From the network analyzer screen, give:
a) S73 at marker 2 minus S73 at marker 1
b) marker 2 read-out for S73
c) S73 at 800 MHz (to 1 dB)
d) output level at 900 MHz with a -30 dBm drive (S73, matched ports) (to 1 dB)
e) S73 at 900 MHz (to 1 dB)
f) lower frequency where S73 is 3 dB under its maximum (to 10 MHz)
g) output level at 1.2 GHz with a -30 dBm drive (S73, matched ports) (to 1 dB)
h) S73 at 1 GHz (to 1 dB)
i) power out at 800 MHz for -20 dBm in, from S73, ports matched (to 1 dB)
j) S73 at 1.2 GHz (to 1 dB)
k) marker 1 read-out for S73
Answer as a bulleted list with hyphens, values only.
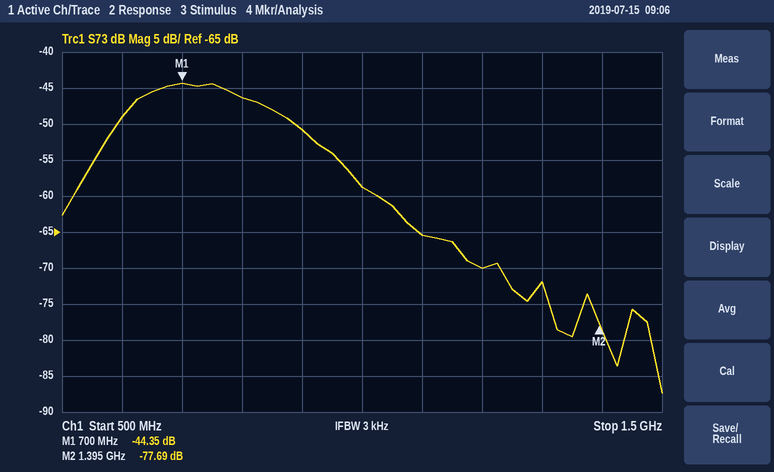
- -33.34 dB
- -77.69 dB
- -46 dB
- -81 dBm
- -51 dB
- 620 MHz
- -100 dBm
- -59 dB
- -66 dBm
- -70 dB
- -44.35 dB
